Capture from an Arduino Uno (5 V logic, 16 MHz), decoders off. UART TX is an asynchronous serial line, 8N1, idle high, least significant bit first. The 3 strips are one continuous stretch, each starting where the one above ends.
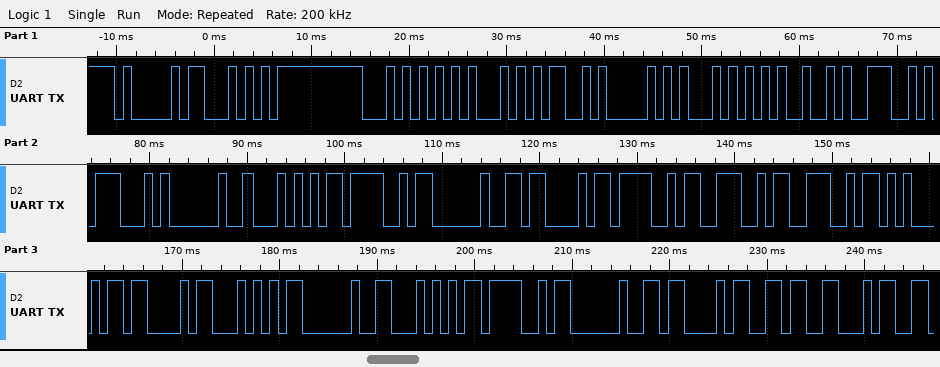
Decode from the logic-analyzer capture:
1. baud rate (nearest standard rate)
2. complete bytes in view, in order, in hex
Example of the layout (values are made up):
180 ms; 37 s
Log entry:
1200 baud; 41 54 54 45 4D 50 54 49 4E 47 20 54 4F 20 43 4F 4E 4E 45 43 54 20 54 4F 20 43 36 34
